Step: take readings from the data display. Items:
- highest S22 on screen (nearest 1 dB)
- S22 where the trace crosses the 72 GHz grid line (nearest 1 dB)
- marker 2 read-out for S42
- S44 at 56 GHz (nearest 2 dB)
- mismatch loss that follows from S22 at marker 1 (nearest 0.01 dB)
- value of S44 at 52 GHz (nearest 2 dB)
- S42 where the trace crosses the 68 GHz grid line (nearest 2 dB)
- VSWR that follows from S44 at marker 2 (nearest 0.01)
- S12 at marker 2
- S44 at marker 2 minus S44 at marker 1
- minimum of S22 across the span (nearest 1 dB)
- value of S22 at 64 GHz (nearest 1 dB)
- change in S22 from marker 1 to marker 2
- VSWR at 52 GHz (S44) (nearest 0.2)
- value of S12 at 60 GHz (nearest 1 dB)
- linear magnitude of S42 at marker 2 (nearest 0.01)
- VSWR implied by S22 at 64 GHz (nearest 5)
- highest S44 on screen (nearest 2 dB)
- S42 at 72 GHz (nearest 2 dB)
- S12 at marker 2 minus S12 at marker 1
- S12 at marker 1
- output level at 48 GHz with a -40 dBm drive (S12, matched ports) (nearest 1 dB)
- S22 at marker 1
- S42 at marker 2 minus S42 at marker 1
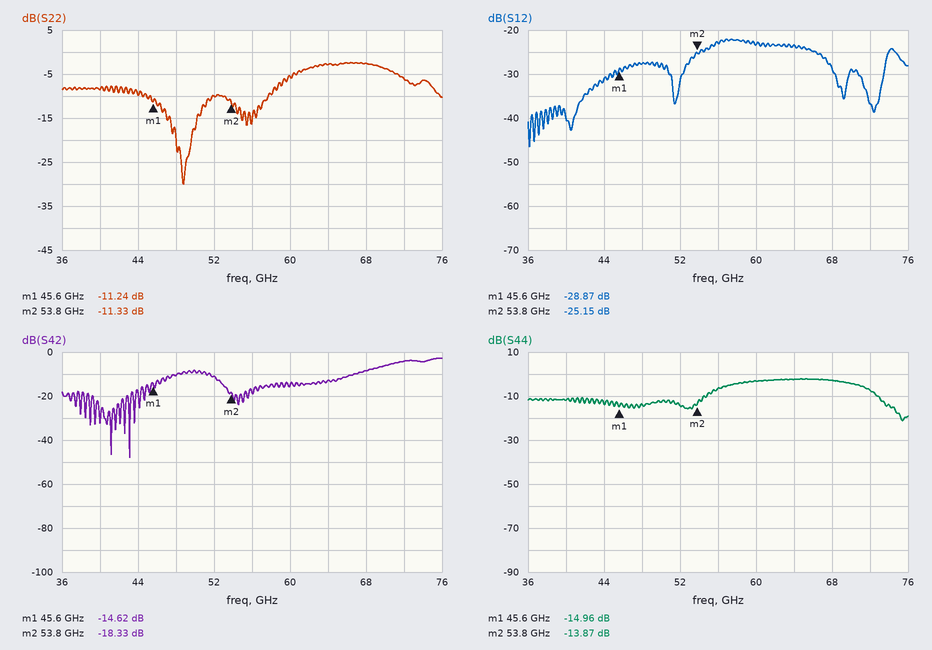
-2 dB
-6 dB
-18.33 dB
-6 dB
0.34 dB
-14 dB
-8 dB
1.51
-25.15 dB
1.09 dB
-30 dB
-3 dB
-0.09 dB
1.4
-23 dB
0.12
5
-2 dB
-4 dB
3.72 dB
-28.87 dB
-68 dBm
-11.24 dB
-3.71 dB
